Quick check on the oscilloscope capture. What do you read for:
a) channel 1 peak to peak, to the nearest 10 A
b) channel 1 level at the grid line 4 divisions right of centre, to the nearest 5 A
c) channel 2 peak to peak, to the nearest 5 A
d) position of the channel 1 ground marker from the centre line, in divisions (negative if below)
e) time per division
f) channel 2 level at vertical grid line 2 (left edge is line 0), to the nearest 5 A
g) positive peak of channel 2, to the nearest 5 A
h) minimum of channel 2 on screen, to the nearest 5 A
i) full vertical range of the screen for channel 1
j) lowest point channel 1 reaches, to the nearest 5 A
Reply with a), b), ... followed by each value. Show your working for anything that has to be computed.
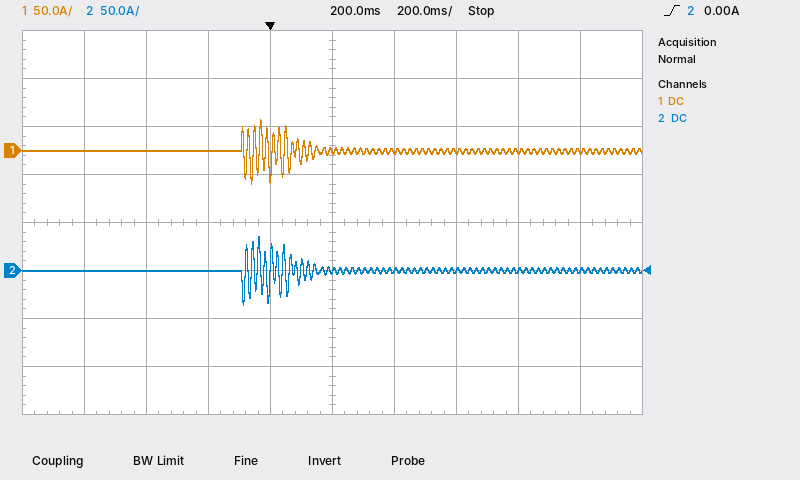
a) 70 A
b) 0 A
c) 35 A − (-35 A) = 70 A
d) +1.5 div
e) 200 ms
f) 0 A
g) 35 A
h) -35 A
i) 400 A
j) -35 A
